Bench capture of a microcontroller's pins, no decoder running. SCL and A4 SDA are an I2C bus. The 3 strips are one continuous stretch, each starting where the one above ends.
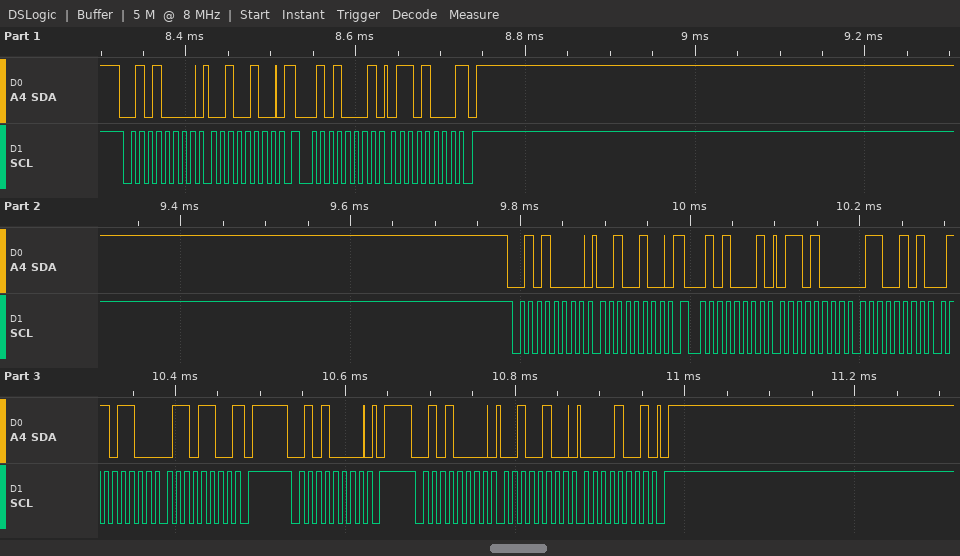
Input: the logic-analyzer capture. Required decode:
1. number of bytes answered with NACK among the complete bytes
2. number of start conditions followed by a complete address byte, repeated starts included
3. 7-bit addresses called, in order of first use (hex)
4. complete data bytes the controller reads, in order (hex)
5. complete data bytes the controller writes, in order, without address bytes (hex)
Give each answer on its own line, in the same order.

2
6
0x28
68 68 65 6C 6C
24 24 24 09
